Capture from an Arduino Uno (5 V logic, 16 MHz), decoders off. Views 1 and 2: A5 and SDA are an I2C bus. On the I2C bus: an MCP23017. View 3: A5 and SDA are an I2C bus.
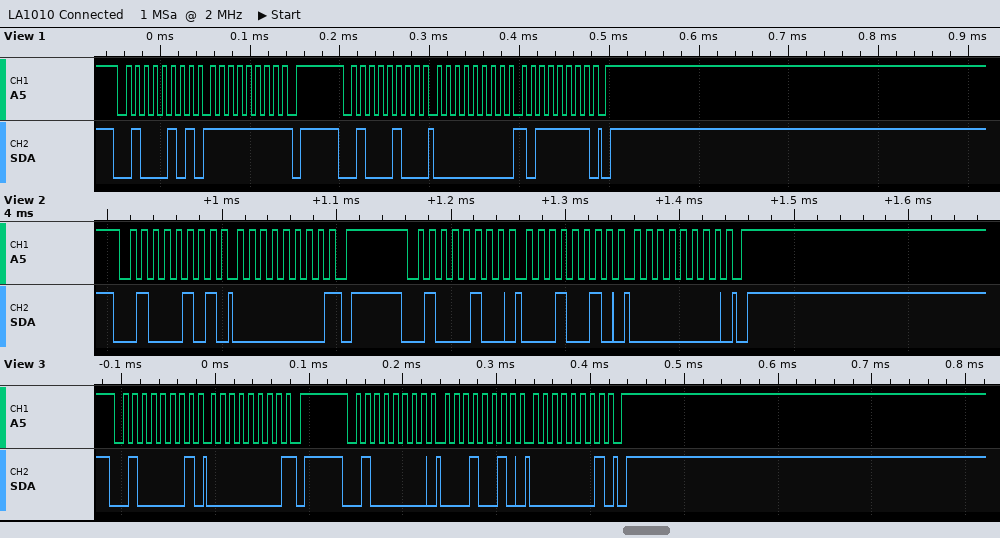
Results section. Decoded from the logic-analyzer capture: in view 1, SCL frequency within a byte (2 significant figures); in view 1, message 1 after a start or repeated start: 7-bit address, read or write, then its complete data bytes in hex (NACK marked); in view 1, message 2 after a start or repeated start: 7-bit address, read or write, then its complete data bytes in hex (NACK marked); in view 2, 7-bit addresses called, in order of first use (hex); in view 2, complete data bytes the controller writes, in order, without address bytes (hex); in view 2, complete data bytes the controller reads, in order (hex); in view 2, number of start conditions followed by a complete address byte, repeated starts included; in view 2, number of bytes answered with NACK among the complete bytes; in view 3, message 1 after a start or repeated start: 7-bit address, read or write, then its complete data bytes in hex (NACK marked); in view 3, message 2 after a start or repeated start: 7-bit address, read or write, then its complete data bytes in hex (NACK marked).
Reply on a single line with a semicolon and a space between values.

100 kHz; 0x22 read: FF NACK; 0x22 write: 00 BF; 0x22; 12 00; 00; 2; 1; 0x20 read: 00 NACK; 0x20 write: 12 01
